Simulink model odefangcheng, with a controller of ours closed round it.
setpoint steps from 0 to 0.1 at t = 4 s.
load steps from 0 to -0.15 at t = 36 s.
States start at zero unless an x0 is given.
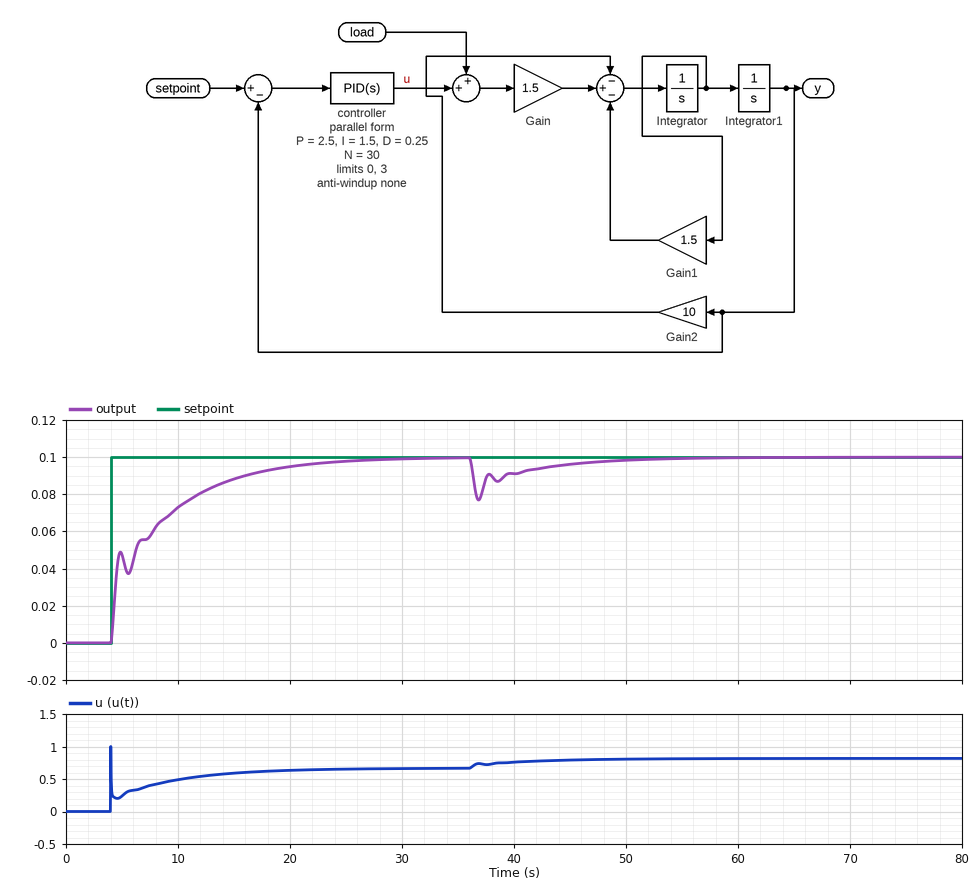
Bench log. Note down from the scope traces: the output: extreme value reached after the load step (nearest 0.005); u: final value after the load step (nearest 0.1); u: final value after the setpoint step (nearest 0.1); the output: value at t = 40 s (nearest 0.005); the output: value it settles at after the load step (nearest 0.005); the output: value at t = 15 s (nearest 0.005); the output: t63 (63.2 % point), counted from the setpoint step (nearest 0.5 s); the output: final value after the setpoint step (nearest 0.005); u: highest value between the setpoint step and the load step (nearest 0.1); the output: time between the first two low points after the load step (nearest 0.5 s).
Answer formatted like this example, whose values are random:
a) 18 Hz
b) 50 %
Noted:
a) 0.075
b) 0.8
c) 0.7
d) 0.090
e) 0.100
f) 0.090
g) 4.0 s
h) 0.100
i) 1.0
j) 1.5 s
